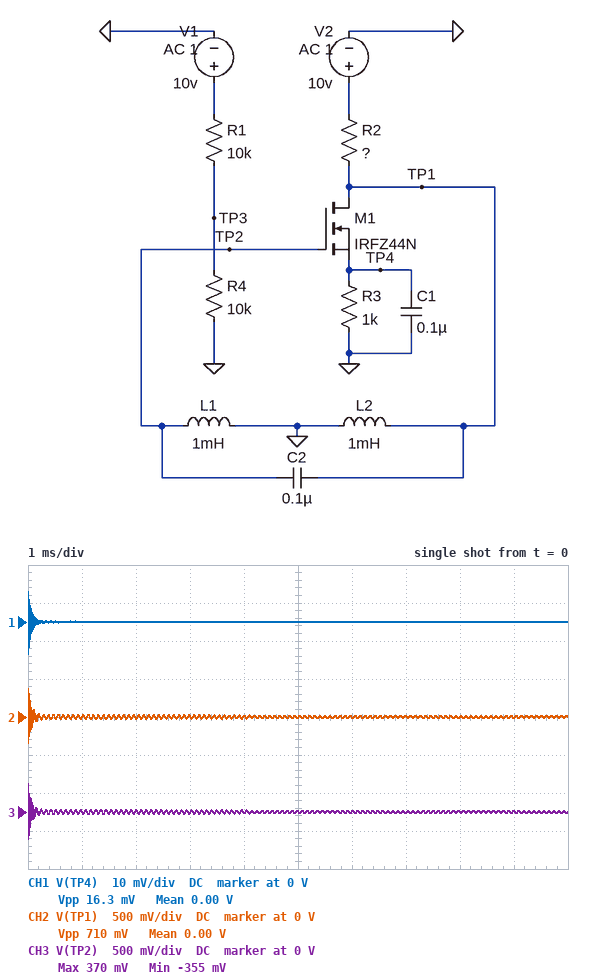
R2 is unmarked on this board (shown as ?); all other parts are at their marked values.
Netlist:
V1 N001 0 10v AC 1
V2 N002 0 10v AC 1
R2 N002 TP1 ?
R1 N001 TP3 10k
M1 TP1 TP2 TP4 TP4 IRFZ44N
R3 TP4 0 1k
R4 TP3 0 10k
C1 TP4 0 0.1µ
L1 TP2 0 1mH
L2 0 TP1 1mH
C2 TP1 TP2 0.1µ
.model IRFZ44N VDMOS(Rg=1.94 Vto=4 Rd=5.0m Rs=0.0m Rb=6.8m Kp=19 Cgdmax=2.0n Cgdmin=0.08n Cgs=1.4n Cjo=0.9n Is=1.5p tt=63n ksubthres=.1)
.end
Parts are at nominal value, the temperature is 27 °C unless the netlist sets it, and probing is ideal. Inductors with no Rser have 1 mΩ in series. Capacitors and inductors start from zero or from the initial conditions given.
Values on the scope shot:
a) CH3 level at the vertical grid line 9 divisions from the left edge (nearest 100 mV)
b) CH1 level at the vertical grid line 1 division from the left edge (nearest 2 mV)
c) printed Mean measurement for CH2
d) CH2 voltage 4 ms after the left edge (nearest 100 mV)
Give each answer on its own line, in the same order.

0 V
0 V
0.00 V
0 V
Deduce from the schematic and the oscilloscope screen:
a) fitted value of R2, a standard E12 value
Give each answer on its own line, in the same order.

12 kΩ
